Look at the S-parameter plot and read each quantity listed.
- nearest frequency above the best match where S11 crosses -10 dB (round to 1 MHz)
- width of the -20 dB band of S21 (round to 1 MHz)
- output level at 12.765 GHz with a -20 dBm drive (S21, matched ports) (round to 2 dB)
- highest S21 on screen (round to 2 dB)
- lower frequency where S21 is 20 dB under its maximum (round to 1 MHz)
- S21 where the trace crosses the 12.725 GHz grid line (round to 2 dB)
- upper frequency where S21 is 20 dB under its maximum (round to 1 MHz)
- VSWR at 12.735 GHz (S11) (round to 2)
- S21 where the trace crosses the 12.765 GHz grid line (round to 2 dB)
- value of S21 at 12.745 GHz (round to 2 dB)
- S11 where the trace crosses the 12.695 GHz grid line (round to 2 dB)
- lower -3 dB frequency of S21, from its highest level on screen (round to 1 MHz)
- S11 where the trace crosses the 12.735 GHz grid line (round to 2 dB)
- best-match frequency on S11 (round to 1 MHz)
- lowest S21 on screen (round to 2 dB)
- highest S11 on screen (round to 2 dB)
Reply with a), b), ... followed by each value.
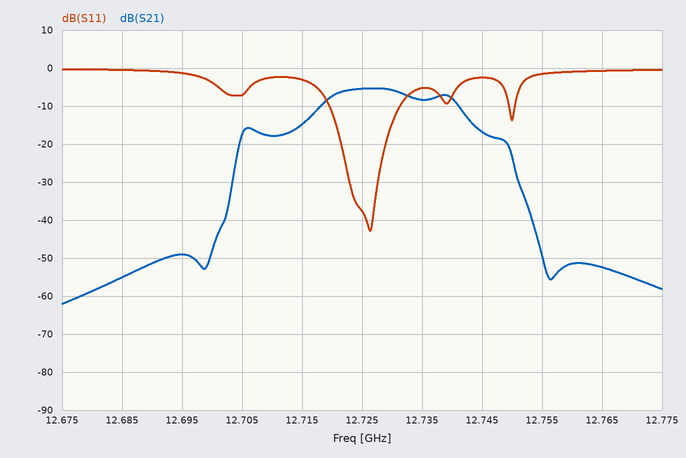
a) 12.731 GHz
b) 46 MHz
c) -72 dBm
d) -6 dB
e) 12.704 GHz
f) -6 dB
g) 12.750 GHz
h) 4
i) -52 dB
j) -16 dB
k) -2 dB
l) 12.719 GHz
m) -6 dB
n) 12.726 GHz
o) -62 dB
p) 0 dB
